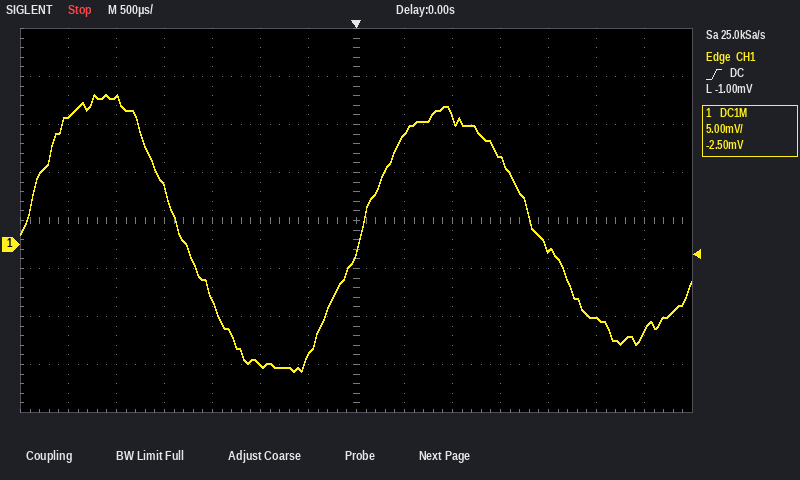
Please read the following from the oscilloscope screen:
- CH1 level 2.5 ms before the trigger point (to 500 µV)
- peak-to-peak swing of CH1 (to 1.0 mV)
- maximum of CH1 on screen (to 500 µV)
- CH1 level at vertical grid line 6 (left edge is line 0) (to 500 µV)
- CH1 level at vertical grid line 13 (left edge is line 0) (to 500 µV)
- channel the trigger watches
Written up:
15.5 mV
29.0 mV
15.5 mV
-11.5 mV
-9.0 mV
CH1
